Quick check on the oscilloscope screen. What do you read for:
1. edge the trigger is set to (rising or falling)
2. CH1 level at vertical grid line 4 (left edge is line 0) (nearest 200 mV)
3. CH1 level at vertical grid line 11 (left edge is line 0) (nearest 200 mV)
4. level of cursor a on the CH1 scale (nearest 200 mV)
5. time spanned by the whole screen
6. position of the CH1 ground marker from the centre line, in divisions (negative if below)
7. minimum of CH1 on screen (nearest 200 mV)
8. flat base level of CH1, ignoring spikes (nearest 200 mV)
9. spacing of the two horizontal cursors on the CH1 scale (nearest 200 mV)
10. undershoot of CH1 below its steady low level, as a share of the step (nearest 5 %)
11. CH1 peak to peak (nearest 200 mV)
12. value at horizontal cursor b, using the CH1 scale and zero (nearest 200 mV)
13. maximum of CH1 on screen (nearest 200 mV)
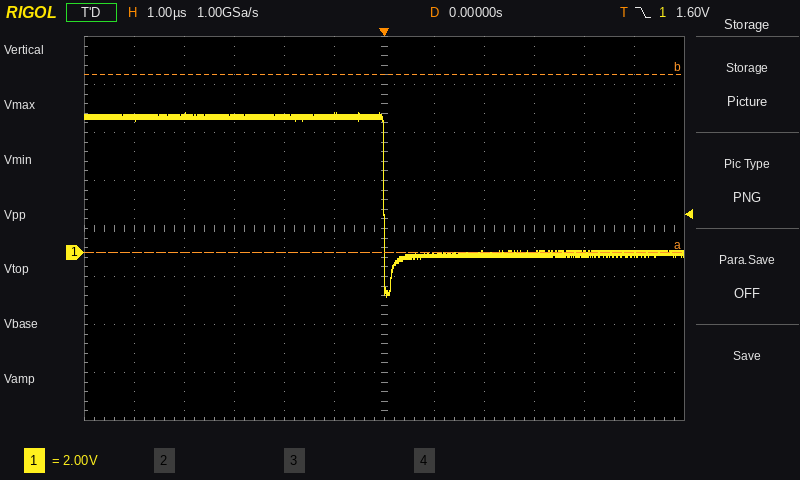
falling
5.6 V
0.0 V
0.0 V
12 µs
-0.5 div
-1.8 V
0.0 V
7.4 V
30 %
7.6 V
7.4 V
5.8 V
